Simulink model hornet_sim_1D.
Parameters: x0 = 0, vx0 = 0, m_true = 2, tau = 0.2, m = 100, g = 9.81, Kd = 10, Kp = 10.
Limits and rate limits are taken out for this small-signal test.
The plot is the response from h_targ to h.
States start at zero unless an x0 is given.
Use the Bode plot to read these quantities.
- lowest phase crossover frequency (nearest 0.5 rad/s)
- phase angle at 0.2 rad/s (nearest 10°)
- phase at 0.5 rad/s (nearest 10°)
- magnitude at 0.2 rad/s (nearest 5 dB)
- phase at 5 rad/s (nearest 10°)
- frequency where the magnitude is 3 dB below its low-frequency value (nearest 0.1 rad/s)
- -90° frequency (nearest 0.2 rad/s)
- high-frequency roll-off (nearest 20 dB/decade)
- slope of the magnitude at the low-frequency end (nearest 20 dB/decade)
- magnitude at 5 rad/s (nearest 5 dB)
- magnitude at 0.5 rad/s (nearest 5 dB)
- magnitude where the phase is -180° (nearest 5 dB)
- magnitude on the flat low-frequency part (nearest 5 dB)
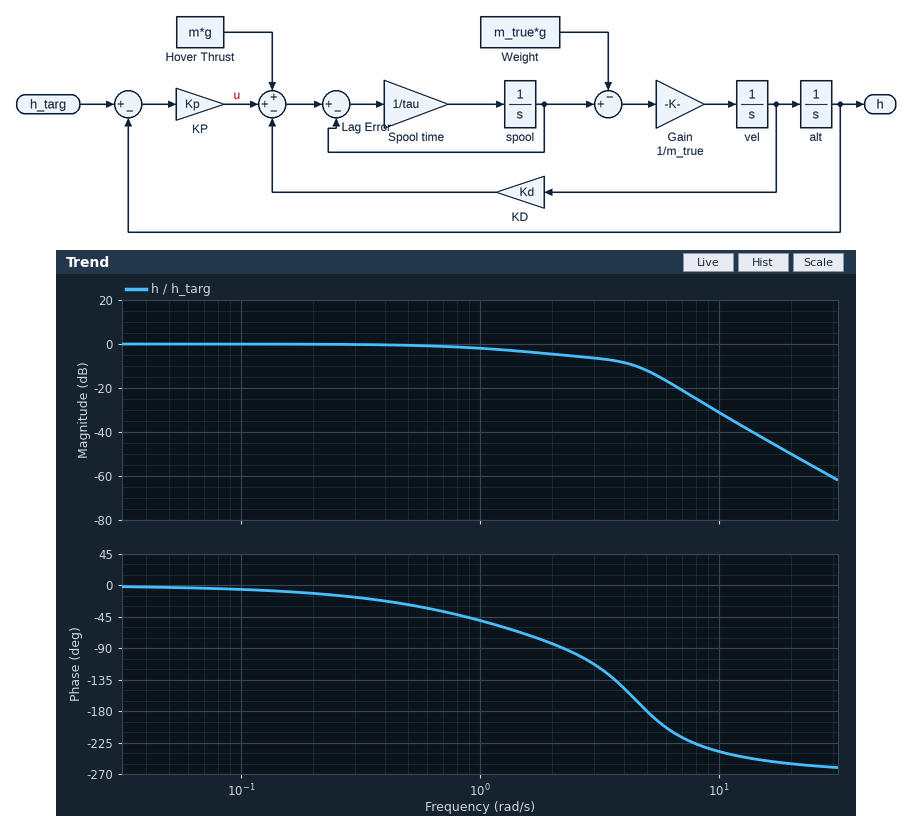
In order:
5.0 rad/s
-10°
-30°
0 dB
-180°
1.4 rad/s
2.2 rad/s
-60 dB/decade
0 dB/decade
-10 dB
0 dB
-10 dB
0 dB
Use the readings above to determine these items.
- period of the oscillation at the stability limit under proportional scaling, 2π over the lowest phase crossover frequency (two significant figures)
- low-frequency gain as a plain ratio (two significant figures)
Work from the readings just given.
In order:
1.3 s
1.0
